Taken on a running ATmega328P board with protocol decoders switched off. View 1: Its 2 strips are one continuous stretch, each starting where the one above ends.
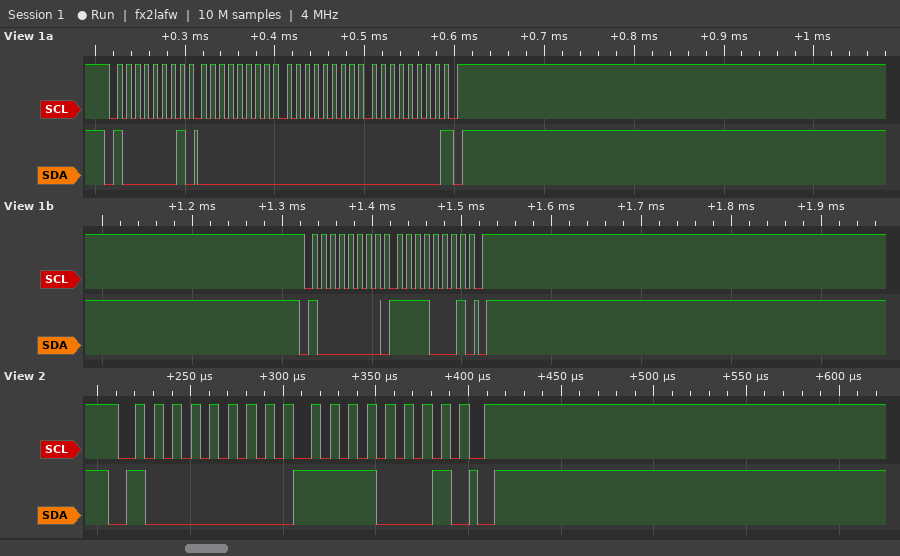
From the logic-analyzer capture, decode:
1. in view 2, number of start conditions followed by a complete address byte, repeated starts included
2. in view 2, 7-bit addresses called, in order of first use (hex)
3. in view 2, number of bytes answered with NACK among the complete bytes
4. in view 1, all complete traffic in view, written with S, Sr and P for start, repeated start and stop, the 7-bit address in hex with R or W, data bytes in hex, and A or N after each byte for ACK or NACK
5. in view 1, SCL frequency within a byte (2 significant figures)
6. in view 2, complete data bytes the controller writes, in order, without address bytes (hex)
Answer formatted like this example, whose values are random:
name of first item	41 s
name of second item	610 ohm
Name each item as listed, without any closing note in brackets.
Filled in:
in view 2, number of start conditions followed by a complete address byte, repeated starts included	1
in view 2, 7-bit addresses called, in order of first use	0x40
in view 2, number of bytes answered with NACK among the complete bytes	0
in view 1, all complete traffic in view, written with S, Sr and P for start, repeated start and stop, the 7-bit address in hex with R or W, data bytes in hex, and A or N after each byte for ACK or NACK	S 40R A 00 A 00 A 00 N P S 40W A F1 A P
in view 1, SCL frequency within a byte	100 kHz
in view 2, complete data bytes the controller writes, in order, without address bytes	F1
